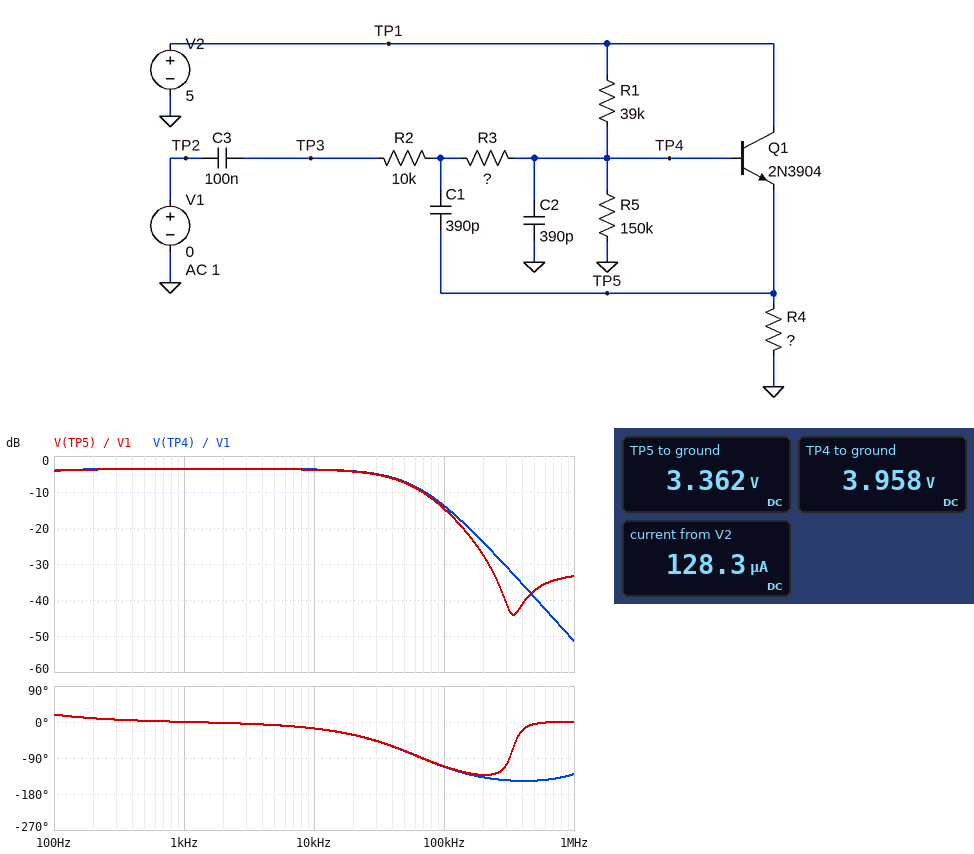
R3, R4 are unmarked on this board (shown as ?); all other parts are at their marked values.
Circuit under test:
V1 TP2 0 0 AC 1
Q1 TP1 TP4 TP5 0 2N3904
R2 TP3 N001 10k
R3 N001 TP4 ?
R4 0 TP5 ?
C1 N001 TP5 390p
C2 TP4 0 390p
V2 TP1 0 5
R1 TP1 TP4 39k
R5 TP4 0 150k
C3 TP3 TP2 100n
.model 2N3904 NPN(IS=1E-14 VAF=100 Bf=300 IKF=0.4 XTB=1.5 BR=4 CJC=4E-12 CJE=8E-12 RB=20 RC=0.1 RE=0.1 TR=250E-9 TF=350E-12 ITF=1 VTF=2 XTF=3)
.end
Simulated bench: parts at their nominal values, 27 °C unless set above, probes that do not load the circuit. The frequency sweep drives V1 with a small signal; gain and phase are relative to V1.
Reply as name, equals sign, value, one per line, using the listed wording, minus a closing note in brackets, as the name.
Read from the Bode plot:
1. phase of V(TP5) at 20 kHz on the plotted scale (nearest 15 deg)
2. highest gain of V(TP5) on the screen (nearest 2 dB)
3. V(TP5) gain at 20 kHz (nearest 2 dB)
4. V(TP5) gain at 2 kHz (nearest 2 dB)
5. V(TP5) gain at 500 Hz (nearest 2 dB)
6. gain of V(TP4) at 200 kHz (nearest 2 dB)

phase of V(TP5) at 20 kHz on the plotted scale = -30 deg
highest gain of V(TP5) on the screen = -4 dB
V(TP5) gain at 20 kHz = -4 dB
V(TP5) gain at 2 kHz = -4 dB
V(TP5) gain at 500 Hz = -4 dB
gain of V(TP4) at 200 kHz = -24 dB
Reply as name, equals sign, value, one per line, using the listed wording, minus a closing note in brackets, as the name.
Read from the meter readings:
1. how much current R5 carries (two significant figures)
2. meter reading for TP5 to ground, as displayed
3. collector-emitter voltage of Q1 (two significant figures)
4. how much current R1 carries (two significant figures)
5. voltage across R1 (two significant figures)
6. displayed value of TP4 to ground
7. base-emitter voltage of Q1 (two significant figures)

how much current R5 carries = 26 µA
meter reading for TP5 to ground, as displayed = 3.362 V
collector-emitter voltage of Q1 = 1.6 V
how much current R1 carries = 27 µA
voltage across R1 = 1.0 V
displayed value of TP4 to ground = 3.958 V
base-emitter voltage of Q1 = 600 mV
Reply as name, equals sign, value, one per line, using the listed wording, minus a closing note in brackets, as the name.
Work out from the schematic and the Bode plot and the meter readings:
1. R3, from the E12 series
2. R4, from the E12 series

R3, from the E12 series = 5.6 kΩ
R4, from the E12 series = 33 kΩ
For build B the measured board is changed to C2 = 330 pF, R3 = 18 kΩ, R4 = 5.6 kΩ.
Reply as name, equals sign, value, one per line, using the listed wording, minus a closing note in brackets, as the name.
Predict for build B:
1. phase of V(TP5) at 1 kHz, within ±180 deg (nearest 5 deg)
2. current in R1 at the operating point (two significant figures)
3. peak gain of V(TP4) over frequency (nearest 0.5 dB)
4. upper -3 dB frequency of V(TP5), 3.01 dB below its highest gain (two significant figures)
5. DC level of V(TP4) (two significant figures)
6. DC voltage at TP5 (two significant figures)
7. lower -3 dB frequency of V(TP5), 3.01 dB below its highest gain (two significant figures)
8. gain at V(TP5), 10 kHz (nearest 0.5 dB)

phase of V(TP5) at 1 kHz, within ±180 deg = 0 deg
current in R1 at the operating point = 28 µA
peak gain of V(TP4) over frequency = -5.5 dB
upper -3 dB frequency of V(TP5), 3.01 dB below its highest gain = 35 kHz
DC level of V(TP4) = 3.9 V
DC voltage at TP5 = 3.3 V
lower -3 dB frequency of V(TP5), 3.01 dB below its highest gain = 27 Hz
gain at V(TP5), 10 kHz = -6.0 dB
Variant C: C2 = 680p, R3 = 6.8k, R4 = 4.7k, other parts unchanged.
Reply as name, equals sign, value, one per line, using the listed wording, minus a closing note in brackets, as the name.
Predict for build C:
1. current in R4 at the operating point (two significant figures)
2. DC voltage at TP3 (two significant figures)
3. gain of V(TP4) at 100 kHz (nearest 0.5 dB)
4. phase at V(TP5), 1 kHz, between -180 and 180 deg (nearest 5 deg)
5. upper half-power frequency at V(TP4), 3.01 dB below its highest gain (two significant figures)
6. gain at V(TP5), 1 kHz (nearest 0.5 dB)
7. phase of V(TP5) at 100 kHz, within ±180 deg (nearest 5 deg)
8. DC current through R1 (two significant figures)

current in R4 at the operating point = 690 µA
DC voltage at TP3 = 3.9 V
gain of V(TP4) at 100 kHz = -19.5 dB
phase at V(TP5), 1 kHz, between -180 and 180 deg = 0 deg
upper half-power frequency at V(TP4), 3.01 dB below its highest gain = 24 kHz
gain at V(TP5), 1 kHz = -4.0 dB
phase of V(TP5) at 100 kHz, within ±180 deg = -125 deg
DC current through R1 = 28 µA
